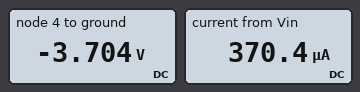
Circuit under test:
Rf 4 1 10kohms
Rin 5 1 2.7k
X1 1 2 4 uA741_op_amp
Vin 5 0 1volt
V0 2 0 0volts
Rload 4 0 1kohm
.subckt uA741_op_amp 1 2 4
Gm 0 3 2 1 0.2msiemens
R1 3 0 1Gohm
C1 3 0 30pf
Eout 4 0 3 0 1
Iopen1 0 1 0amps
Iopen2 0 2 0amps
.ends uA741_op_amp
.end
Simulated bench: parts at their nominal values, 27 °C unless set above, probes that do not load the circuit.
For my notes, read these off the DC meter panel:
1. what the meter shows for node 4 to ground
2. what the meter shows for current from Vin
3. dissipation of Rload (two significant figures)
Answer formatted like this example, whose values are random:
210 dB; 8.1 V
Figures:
-3.704 V; 370.4 µA; 14 mW
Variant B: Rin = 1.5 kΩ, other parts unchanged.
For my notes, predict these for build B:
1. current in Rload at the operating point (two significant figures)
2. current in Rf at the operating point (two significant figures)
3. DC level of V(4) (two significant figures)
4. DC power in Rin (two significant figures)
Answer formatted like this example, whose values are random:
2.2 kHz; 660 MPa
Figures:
6.7 mA; 670 µA; -6.7 V; 670 µW
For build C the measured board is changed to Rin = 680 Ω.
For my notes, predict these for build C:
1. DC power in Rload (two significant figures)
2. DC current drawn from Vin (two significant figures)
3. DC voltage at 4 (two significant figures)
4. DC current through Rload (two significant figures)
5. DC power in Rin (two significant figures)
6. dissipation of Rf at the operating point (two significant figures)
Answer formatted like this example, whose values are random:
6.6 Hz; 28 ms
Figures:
220 mW; 1.5 mA; -15 V; 15 mA; 1.5 mW; 22 mW
